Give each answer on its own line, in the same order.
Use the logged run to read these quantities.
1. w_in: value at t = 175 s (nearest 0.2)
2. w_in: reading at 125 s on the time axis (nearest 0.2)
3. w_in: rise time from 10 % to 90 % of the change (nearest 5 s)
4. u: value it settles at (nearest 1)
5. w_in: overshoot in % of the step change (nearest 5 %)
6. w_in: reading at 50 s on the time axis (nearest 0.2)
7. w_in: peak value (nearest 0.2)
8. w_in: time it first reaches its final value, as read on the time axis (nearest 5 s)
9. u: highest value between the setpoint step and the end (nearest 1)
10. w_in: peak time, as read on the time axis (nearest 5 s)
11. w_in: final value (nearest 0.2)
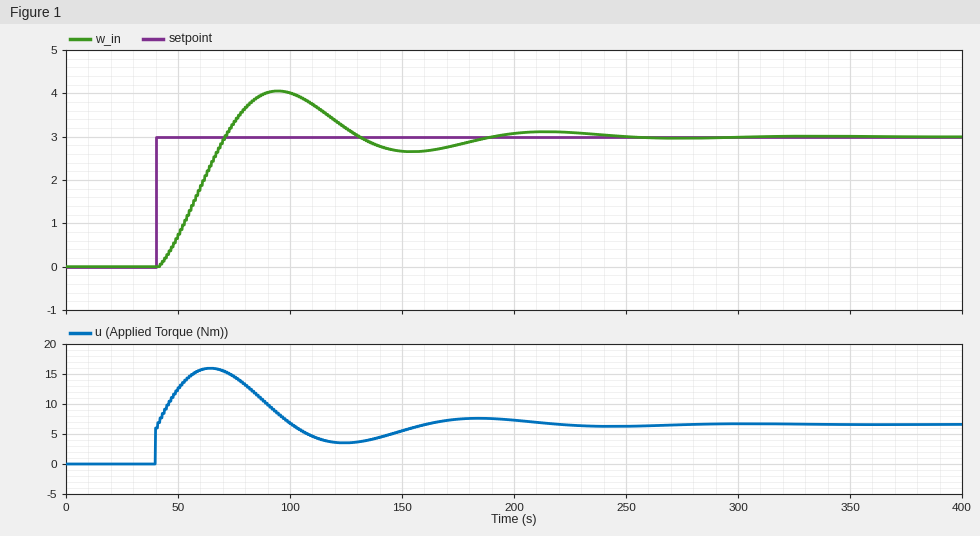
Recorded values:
2.8
3.2
20 s
7
35 %
0.8
4.0
70 s
16
95 s
3.0
